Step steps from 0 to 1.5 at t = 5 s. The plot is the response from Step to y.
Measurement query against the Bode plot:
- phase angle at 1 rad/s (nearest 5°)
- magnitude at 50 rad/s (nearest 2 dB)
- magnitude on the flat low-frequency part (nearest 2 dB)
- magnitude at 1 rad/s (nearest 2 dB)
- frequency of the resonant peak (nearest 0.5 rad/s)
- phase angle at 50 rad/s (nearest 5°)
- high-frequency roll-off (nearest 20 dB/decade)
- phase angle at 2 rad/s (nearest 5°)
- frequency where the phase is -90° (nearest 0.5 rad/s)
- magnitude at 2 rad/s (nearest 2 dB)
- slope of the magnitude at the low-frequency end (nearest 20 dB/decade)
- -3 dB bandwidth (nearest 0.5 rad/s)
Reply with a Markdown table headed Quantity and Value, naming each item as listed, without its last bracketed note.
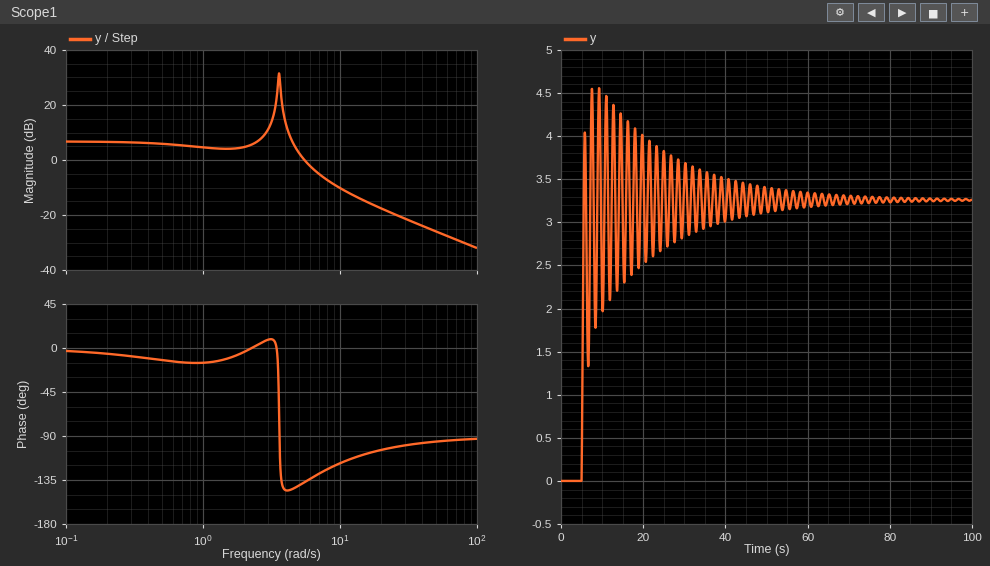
| Quantity | Value |
|---|---|
| phase angle at 1 rad/s | -15° |
| magnitude at 50 rad/s | -26 dB |
| magnitude on the flat low-frequency part | 6 dB |
| magnitude at 1 rad/s | 4 dB |
| frequency of the resonant peak | 3.5 rad/s |
| phase angle at 50 rad/s | -95° |
| high-frequency roll-off | -20 dB/decade |
| phase angle at 2 rad/s | -5° |
| frequency where the phase is -90° | 3.5 rad/s |
| magnitude at 2 rad/s | 4 dB |
| slope of the magnitude at the low-frequency end | 0 dB/decade |
| -3 dB bandwidth | 5.0 rad/s |
